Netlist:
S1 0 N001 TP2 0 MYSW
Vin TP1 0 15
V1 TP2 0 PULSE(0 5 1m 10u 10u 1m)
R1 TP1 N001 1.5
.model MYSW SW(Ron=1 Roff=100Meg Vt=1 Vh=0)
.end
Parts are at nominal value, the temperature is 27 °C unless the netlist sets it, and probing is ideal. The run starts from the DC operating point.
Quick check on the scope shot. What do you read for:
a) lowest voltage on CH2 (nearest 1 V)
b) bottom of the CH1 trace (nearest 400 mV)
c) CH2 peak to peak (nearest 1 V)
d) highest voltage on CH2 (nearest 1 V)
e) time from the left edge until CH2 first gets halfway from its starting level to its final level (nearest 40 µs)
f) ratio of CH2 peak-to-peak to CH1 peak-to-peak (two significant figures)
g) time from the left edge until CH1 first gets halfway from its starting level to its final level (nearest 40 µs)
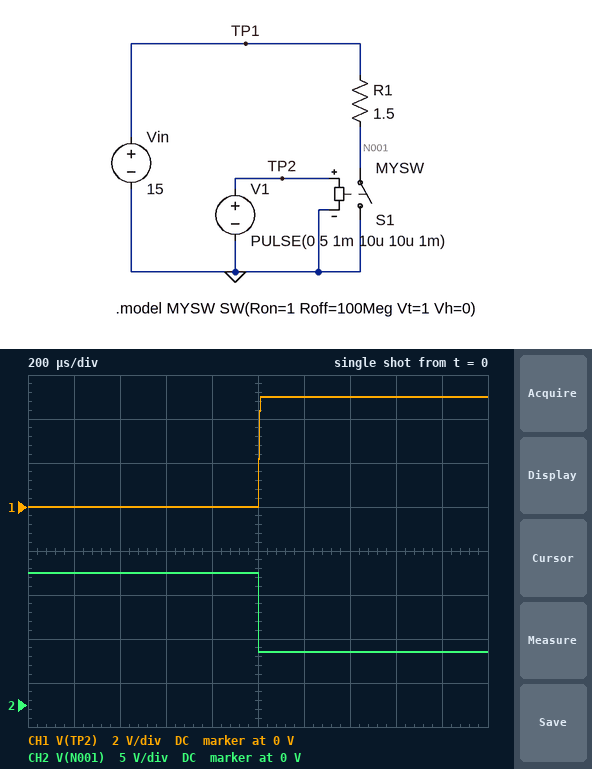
6 V
0 V
9 V
15 V
1.00 ms
1.8
1.00 ms
